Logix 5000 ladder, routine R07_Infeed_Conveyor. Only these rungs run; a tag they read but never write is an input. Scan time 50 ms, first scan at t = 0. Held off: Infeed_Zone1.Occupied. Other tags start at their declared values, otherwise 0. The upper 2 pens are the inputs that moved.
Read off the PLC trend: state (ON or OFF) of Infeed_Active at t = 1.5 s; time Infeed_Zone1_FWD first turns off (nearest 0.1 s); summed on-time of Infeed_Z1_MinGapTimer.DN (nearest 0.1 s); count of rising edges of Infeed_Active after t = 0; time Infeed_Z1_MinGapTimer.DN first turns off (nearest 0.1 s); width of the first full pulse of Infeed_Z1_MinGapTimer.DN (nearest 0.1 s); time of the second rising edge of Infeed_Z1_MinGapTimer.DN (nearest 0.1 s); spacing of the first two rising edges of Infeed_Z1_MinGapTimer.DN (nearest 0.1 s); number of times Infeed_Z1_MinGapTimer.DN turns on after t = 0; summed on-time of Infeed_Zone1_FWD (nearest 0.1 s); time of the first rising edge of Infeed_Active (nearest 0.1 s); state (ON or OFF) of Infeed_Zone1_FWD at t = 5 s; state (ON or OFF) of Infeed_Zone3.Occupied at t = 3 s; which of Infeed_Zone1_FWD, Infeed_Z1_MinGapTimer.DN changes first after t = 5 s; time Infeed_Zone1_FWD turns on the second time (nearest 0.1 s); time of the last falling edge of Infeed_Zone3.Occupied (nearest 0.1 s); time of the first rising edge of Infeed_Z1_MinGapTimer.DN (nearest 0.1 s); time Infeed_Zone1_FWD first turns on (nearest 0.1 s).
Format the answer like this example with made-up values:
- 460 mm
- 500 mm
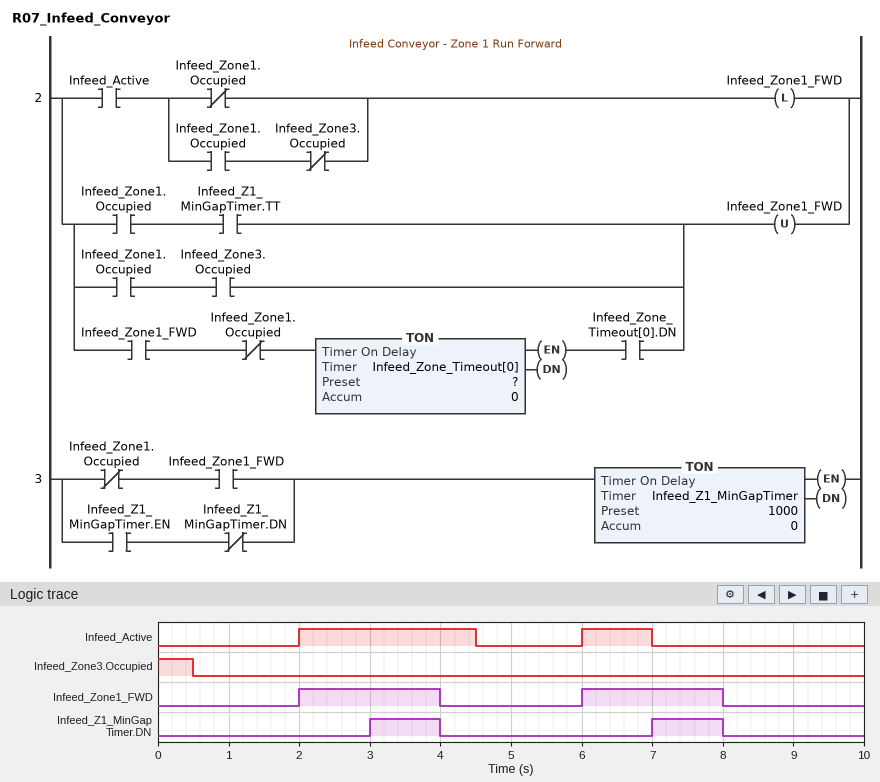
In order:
- OFF
- 4.0 s
- 2.0 s
- 2
- 4.0 s
- 1.0 s
- 7.0 s
- 4.0 s
- 2
- 4.0 s
- 2.0 s
- OFF
- OFF
- Infeed_Zone1_FWD
- 6.0 s
- 0.5 s
- 3.0 s
- 2.0 s
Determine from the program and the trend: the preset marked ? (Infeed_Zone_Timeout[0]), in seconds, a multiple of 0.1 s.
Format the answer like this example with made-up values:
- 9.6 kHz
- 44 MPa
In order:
- 2.0 s
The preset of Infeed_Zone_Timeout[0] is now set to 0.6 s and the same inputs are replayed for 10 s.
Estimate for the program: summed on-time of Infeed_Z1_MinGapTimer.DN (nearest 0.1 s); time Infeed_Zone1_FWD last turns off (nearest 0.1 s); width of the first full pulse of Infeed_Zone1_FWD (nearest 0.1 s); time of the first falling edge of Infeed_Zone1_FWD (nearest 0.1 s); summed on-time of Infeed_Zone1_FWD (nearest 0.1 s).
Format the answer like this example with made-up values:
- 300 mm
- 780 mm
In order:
- 0.1 s
- 6.6 s
- 0.6 s
- 2.6 s
- 1.2 s
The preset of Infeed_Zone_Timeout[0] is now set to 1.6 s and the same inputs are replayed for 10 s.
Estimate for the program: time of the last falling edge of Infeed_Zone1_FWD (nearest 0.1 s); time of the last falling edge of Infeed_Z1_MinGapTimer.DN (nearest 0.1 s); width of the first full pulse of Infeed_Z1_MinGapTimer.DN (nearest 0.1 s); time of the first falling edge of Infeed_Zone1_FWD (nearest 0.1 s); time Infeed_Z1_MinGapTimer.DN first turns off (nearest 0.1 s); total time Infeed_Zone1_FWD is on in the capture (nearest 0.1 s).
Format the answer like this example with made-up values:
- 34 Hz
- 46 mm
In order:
- 7.6 s
- 7.6 s
- 0.6 s
- 3.6 s
- 3.6 s
- 3.2 s
